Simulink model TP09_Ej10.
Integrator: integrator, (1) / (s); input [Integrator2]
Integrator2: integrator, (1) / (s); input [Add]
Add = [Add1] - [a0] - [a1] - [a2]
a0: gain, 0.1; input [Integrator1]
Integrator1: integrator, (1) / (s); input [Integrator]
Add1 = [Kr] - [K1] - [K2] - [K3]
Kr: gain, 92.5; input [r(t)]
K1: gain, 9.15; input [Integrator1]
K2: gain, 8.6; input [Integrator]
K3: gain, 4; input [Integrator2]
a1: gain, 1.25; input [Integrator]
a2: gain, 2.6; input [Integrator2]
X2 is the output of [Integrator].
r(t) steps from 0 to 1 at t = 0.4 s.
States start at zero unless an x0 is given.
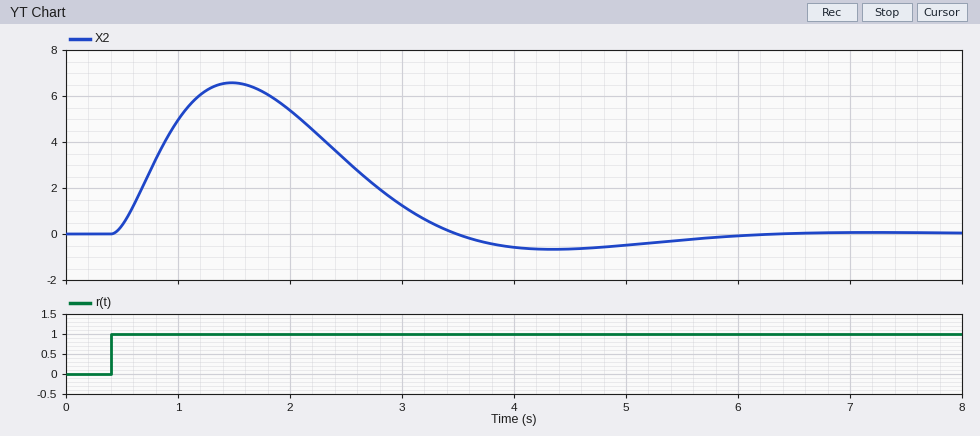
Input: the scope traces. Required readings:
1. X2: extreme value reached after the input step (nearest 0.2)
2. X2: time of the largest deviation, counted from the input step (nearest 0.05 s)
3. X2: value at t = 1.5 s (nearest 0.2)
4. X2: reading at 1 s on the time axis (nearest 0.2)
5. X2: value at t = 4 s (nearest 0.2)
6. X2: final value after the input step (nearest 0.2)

6.6
1.10 s
6.6
5.0
-0.6
0.0
